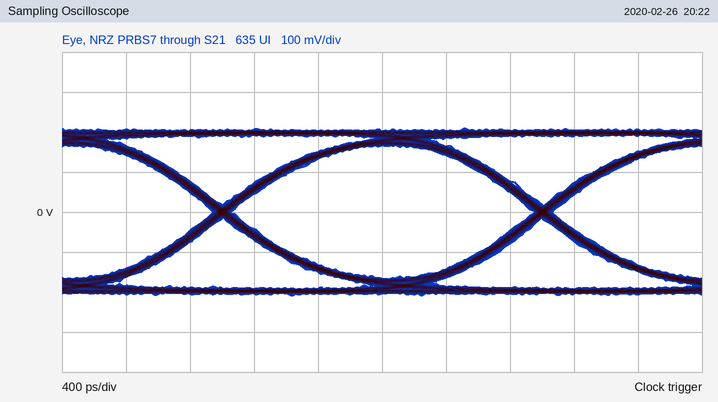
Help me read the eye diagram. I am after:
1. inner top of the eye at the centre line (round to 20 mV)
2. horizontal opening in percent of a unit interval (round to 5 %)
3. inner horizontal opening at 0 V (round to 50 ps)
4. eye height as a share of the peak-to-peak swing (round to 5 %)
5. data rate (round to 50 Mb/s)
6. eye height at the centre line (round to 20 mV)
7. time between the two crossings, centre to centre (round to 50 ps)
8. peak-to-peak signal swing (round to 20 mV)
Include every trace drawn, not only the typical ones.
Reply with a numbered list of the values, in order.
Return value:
1. 160 mV
2. 95 %
3. 1.90 ns
4. 80 %
5. 500 Mb/s
6. 340 mV
7. 2.00 ns
8. 420 mV
